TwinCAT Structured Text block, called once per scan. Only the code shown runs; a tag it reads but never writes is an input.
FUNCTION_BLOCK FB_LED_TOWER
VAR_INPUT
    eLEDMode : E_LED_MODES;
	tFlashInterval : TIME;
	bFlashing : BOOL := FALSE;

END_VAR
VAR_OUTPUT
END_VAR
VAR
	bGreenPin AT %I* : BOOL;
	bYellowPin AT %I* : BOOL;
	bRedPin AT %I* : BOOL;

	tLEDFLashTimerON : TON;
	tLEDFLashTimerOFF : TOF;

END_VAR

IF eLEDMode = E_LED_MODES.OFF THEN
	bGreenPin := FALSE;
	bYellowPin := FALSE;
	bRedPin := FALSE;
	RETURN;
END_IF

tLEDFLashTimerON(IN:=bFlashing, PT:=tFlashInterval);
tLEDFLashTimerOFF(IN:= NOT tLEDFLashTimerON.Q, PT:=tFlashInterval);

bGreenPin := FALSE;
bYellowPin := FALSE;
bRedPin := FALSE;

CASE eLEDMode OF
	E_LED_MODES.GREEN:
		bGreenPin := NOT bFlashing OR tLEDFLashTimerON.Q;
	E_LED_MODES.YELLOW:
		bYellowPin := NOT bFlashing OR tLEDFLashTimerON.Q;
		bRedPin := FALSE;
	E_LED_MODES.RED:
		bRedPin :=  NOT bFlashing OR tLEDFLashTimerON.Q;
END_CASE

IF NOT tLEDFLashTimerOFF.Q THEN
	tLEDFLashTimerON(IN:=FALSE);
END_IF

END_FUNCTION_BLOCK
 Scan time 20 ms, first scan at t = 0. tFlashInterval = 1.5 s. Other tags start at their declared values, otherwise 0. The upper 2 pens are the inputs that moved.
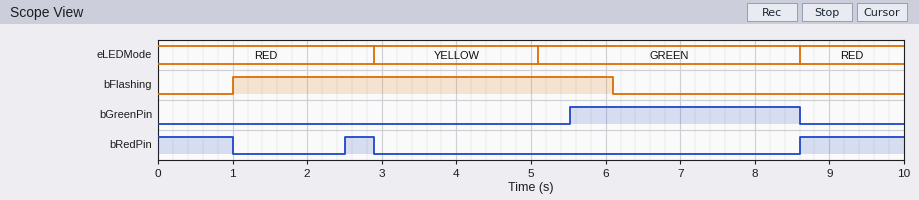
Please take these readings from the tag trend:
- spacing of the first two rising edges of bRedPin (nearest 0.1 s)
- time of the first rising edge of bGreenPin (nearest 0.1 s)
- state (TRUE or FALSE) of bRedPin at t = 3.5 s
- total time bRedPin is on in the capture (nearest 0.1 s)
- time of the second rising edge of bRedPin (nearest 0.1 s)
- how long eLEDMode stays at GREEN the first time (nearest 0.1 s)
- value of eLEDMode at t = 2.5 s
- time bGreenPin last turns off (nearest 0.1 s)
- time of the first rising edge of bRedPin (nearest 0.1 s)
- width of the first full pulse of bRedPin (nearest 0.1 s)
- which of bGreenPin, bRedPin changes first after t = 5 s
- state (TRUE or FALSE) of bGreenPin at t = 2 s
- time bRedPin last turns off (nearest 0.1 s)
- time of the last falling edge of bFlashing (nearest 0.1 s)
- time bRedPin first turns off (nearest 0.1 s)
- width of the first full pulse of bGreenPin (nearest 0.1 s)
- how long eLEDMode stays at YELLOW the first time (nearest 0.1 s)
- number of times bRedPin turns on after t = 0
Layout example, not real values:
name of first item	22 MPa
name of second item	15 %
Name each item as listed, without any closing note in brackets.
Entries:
spacing of the first two rising edges of bRedPin	6.1 s
time of the first rising edge of bGreenPin	5.5 s
state (TRUE or FALSE) of bRedPin at t = 3.5 s	FALSE
total time bRedPin is on in the capture	2.8 s
time of the second rising edge of bRedPin	8.6 s
how long eLEDMode stays at GREEN the first time	3.5 s
value of eLEDMode at t = 2.5 s	RED
time bGreenPin last turns off	8.6 s
time of the first rising edge of bRedPin	2.5 s
width of the first full pulse of bRedPin	0.4 s
which of bGreenPin, bRedPin changes first after t = 5 s	bGreenPin
state (TRUE or FALSE) of bGreenPin at t = 2 s	FALSE
time bRedPin last turns off	2.9 s
time of the last falling edge of bFlashing	6.1 s
time bRedPin first turns off	1.0 s
width of the first full pulse of bGreenPin	3.1 s
how long eLEDMode stays at YELLOW the first time	2.2 s
number of times bRedPin turns on after t = 0	2
